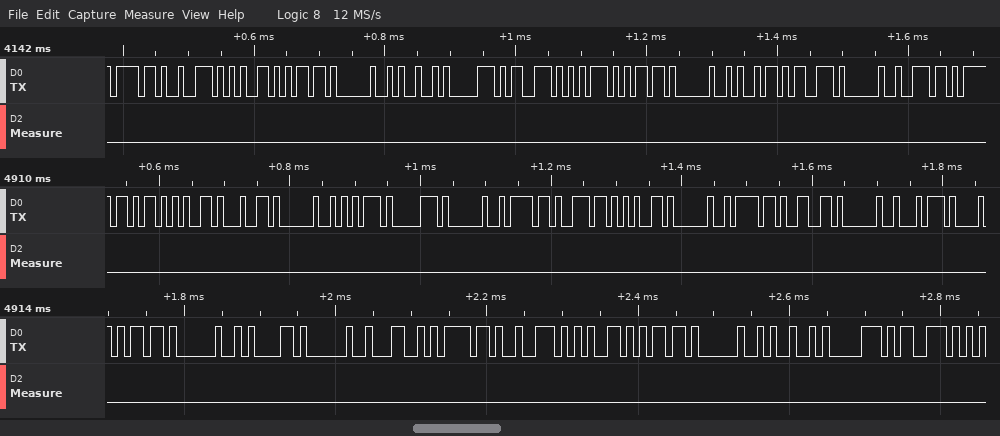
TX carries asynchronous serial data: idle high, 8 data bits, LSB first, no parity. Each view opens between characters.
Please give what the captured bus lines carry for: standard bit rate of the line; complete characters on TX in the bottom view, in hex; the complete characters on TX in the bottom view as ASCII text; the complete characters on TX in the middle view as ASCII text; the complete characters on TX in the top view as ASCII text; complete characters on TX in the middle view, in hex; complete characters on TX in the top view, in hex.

115200 baud
6D, 20, 61, 20, 4C, 6F, 72, 65, 6D, 20, 49, 70, 73
"m a Lorem Ips"
"ked up one of t"
"orem Ipsum is n"
6B, 65, 64, 20, 75, 70, 20, 6F, 6E, 65, 20, 6F, 66, 20, 74
6F, 72, 65, 6D, 20, 49, 70, 73, 75, 6D, 20, 69, 73, 20, 6E
